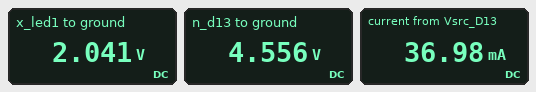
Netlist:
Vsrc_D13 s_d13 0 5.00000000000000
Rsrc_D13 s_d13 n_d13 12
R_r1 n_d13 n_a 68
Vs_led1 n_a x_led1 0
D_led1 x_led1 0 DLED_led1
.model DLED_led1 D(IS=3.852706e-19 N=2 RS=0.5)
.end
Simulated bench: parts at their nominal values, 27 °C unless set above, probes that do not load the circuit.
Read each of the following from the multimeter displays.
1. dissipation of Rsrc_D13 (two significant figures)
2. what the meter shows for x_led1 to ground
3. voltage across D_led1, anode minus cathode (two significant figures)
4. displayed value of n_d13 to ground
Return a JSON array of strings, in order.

["16 mW", "2.041 V", "2.0 V", "4.556 V"]
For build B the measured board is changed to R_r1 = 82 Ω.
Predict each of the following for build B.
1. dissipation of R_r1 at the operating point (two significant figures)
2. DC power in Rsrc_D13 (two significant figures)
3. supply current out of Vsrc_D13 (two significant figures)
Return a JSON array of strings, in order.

["82 mW", "12 mW", "32 mA"]
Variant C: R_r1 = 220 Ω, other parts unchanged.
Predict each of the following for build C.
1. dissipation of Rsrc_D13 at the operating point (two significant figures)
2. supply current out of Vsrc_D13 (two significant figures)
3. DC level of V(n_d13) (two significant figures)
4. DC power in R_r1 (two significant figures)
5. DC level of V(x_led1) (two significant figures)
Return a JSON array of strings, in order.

["2.0 mW", "13 mA", "4.8 V", "37 mW", "2.0 V"]
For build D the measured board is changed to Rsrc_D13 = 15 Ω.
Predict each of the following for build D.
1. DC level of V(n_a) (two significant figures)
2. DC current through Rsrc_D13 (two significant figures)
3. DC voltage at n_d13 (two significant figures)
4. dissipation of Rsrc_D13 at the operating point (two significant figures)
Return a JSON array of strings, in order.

["2.0 V", "36 mA", "4.5 V", "19 mW"]
